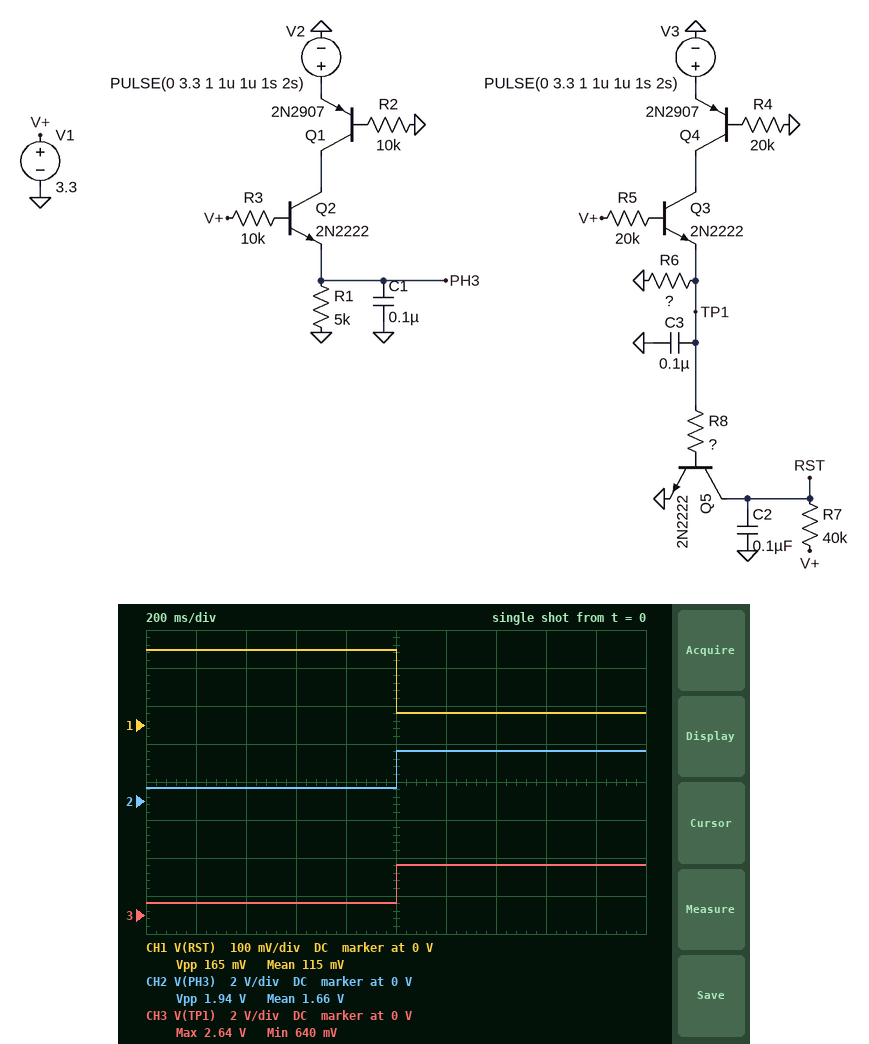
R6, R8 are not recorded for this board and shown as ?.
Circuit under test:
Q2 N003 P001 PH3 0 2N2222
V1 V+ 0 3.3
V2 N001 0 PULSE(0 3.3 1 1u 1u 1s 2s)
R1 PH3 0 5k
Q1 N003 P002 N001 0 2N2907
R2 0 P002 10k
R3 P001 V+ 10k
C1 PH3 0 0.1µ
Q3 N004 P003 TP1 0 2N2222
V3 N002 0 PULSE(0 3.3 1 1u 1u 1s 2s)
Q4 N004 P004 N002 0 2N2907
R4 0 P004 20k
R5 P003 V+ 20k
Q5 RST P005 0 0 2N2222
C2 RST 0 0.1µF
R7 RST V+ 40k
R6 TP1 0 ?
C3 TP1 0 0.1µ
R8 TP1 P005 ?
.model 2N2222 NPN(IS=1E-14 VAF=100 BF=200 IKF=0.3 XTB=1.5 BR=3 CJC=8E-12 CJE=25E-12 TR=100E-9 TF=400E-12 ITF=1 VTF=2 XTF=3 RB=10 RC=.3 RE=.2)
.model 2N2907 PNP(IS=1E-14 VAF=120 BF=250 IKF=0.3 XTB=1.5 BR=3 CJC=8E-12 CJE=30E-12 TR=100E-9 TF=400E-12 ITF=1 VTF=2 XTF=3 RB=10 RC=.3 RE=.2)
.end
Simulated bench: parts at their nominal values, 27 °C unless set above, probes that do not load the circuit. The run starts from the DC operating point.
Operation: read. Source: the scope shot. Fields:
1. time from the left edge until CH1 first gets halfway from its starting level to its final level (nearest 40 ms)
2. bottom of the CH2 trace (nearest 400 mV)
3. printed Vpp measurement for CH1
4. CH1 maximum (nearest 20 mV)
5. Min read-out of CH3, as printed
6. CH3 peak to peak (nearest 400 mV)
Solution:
1.00 s
800 mV
165 mV
200 mV
640 mV
2.0 V
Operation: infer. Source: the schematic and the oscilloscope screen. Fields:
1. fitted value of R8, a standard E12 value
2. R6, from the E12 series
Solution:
150 kΩ
8.2 kΩ
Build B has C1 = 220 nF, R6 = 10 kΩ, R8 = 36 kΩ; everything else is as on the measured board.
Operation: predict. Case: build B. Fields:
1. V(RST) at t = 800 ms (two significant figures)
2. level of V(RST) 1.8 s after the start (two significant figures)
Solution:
68 mV
16 mV
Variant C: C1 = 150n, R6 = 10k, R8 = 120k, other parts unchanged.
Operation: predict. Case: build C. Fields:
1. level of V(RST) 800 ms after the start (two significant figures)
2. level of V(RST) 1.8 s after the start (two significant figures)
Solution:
110 mV
29 mV
